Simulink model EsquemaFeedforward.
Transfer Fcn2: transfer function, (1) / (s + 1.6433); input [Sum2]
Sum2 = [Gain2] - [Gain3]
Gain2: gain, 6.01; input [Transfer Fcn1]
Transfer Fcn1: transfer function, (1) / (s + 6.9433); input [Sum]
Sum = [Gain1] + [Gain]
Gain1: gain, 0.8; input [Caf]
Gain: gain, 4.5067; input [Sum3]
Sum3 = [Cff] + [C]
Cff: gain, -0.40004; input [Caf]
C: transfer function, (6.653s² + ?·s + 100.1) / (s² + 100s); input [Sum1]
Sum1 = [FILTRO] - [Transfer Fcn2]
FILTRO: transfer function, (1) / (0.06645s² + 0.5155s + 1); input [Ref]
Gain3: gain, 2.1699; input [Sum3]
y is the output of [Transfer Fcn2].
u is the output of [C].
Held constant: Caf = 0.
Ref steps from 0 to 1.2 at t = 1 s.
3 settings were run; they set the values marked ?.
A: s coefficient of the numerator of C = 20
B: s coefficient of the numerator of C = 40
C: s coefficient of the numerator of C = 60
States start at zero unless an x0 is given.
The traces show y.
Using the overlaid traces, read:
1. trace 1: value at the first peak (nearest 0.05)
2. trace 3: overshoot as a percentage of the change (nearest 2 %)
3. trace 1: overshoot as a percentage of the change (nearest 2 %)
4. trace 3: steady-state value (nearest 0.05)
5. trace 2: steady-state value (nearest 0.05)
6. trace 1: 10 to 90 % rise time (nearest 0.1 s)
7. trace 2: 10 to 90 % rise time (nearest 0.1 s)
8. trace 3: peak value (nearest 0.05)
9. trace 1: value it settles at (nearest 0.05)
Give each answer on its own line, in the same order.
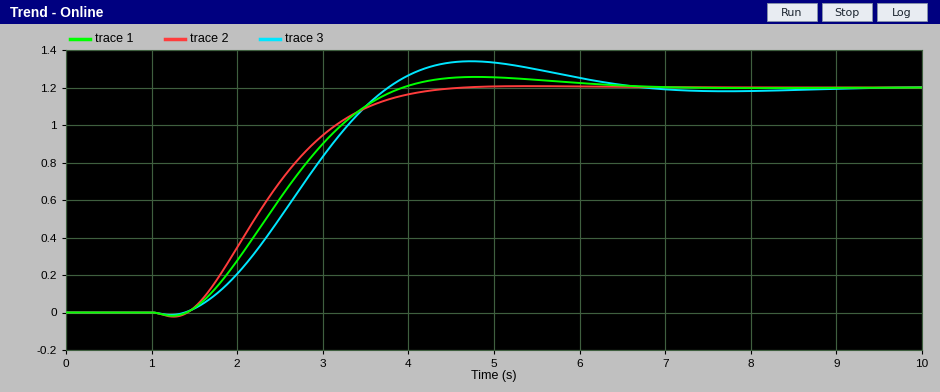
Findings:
1.25
12 %
4 %
1.20
1.20
1.7 s
1.8 s
1.35
1.20
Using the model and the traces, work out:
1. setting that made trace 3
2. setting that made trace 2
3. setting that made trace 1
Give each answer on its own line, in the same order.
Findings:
A
C
B
